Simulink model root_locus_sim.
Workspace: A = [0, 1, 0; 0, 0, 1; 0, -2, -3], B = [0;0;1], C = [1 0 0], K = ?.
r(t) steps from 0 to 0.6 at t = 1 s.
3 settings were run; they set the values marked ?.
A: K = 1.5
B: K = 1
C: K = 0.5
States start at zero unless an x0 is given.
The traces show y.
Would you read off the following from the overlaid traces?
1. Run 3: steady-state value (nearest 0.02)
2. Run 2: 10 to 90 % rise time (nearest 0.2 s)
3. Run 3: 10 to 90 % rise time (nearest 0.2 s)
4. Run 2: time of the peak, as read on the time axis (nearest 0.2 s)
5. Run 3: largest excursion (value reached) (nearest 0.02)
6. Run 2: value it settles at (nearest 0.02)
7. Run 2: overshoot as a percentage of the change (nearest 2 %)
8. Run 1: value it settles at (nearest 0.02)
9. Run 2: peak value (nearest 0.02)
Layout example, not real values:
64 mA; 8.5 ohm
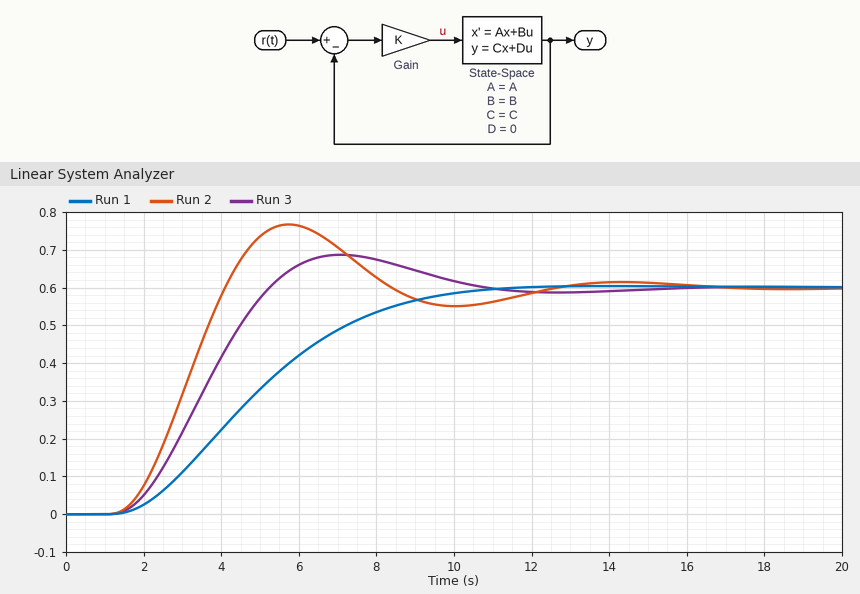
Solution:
0.60; 2.0 s; 2.6 s; 5.8 s; 0.68; 0.60; 28 %; 0.60; 0.76
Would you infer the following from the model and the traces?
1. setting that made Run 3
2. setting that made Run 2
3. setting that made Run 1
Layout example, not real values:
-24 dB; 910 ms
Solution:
B; A; C
